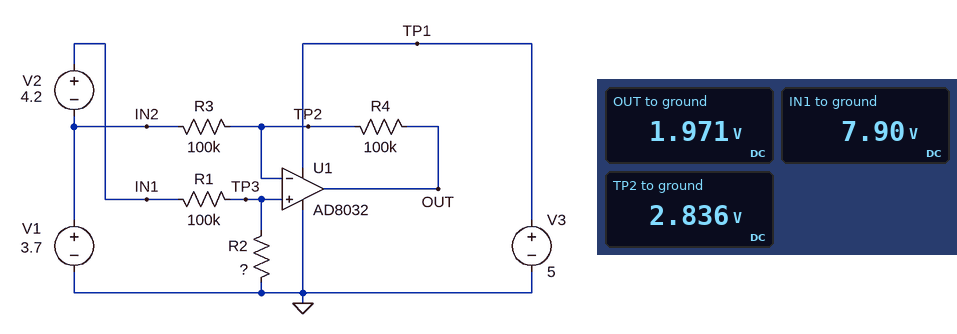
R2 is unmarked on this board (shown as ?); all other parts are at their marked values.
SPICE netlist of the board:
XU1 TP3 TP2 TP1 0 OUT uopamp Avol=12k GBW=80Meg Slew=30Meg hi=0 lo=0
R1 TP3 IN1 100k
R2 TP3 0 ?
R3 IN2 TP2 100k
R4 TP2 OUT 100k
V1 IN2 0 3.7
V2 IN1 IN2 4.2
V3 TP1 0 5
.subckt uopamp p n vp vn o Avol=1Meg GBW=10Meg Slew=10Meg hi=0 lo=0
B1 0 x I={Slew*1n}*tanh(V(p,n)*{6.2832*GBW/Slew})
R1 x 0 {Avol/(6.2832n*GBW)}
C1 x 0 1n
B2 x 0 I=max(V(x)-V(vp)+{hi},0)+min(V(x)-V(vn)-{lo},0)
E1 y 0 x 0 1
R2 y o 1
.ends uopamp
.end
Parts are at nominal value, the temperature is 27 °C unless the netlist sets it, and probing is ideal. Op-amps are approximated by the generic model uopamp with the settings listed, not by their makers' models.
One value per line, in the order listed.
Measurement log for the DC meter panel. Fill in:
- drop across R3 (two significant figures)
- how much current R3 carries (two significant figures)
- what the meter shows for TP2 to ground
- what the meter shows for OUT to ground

860 mV
8.6 µA
2.836 V
1.971 V
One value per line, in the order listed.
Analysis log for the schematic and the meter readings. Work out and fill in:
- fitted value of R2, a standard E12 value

56 kΩ
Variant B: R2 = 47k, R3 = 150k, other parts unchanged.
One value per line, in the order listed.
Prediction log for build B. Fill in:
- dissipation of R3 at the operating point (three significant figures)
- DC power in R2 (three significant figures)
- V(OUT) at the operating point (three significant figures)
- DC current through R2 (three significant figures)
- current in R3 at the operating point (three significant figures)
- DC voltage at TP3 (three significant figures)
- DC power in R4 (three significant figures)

9.19 µW
136 µW
1.74 V
53.7 µA
7.83 µA
2.53 V
6.13 µW
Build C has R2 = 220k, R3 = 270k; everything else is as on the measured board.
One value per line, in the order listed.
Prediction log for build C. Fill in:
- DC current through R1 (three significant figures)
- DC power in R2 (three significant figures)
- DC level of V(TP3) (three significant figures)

24.7 µA
134 µW
5.43 V
